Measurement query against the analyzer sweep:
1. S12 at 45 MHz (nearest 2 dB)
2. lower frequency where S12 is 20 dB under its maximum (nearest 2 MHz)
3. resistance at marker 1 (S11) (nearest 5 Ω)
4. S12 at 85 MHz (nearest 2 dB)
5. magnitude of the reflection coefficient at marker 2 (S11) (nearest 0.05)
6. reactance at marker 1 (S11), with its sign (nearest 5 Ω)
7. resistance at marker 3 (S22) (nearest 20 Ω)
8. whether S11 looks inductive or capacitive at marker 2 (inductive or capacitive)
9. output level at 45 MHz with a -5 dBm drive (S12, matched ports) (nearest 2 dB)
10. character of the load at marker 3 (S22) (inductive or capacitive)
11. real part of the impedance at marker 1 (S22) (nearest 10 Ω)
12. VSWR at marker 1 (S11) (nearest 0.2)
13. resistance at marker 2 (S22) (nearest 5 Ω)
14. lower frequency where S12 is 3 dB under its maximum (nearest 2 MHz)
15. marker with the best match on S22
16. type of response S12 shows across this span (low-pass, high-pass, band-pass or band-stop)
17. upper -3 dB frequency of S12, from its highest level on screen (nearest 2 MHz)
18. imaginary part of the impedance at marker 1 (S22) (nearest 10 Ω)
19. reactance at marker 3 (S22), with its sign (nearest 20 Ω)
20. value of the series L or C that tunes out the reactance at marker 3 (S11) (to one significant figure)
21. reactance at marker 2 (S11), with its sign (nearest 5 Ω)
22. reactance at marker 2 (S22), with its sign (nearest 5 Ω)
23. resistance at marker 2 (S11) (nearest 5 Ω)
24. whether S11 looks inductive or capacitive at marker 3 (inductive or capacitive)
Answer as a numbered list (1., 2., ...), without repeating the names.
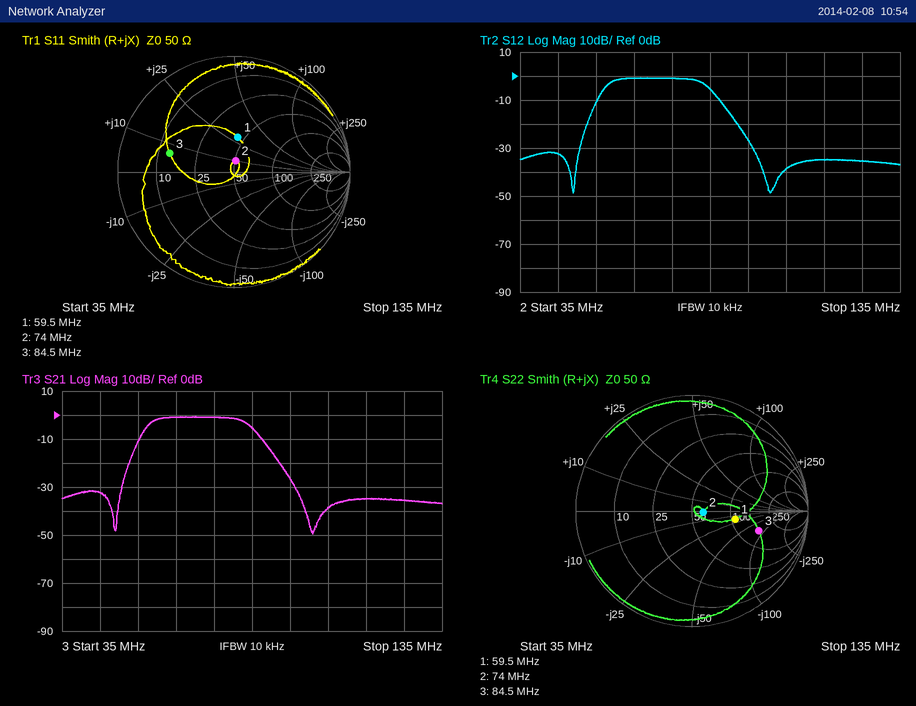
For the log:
1. -32 dB
2. 52 MHz
3. 45 Ω
4. -6 dB
5. 0.10
6. +30 Ω
7. 160 Ω
8. inductive
9. -38 dBm
10. capacitive
11. 110 Ω
12. 1.8
13. 60 Ω
14. 58 MHz
15. marker 2
16. band-pass
17. 84 MHz
18. -20 Ω
19. -80 Ω
20. 300 pF
21. +10 Ω
22. 0 Ω
23. 50 Ω
24. inductive
